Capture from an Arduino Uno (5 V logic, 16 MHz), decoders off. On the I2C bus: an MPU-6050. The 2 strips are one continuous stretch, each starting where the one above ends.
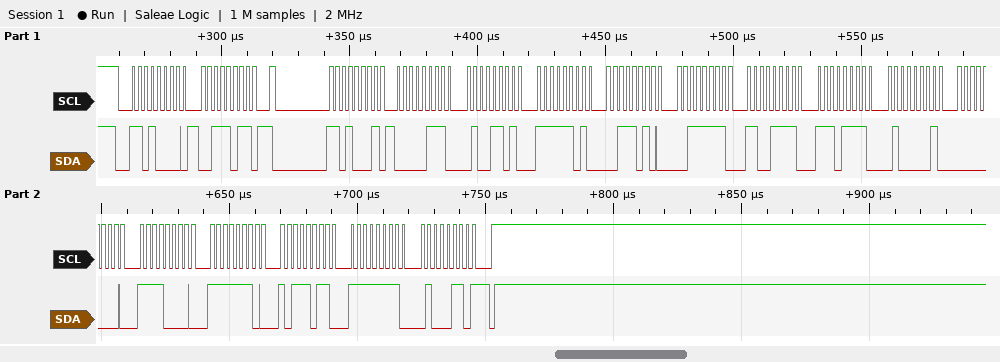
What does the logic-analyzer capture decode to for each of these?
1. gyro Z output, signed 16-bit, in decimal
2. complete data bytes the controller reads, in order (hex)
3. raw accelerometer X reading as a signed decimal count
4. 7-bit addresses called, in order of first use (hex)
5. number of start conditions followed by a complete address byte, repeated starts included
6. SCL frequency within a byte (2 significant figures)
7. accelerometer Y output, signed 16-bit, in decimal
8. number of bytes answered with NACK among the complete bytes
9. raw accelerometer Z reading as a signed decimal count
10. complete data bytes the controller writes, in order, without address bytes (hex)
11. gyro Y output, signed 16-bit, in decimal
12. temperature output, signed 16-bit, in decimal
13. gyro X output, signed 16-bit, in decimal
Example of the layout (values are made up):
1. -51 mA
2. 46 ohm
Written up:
1. -186
2. 07 4D FD 3A 3F CF EF 41 00 F0 FE BB FF 46
3. 1869
4. 0x68
5. 2
6. 400 kHz
7. -710
8. 1
9. 16335
10. 3B
11. -325
12. -4287
13. 240
